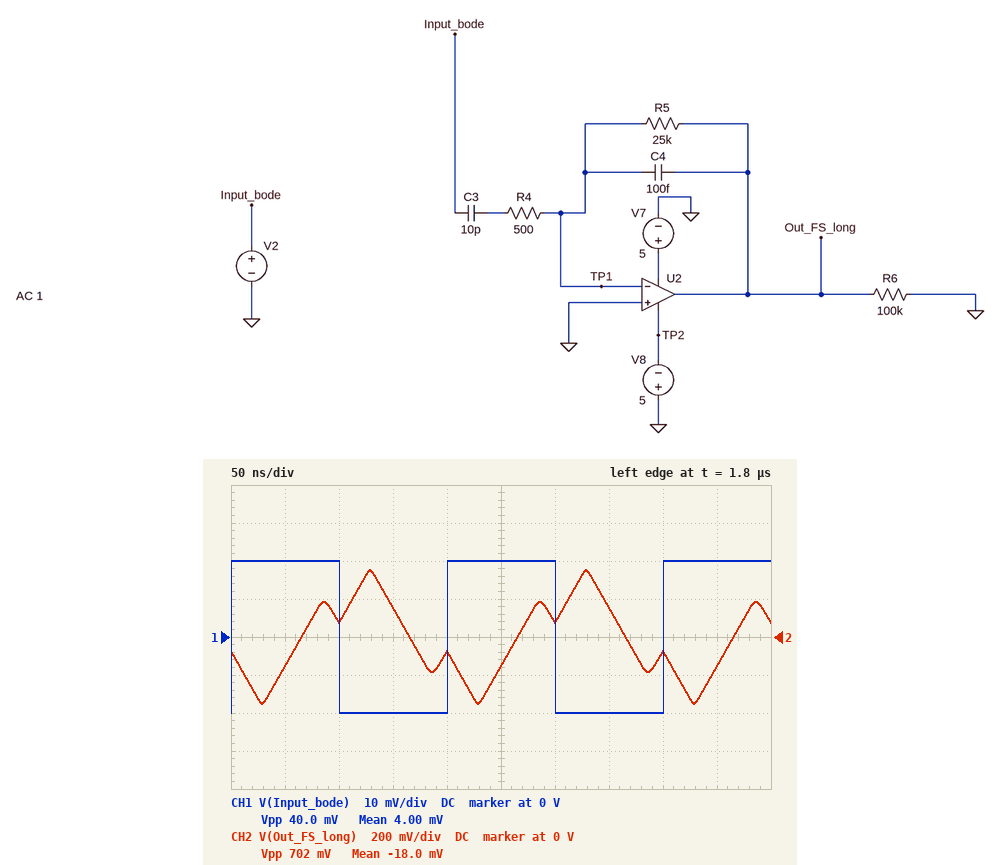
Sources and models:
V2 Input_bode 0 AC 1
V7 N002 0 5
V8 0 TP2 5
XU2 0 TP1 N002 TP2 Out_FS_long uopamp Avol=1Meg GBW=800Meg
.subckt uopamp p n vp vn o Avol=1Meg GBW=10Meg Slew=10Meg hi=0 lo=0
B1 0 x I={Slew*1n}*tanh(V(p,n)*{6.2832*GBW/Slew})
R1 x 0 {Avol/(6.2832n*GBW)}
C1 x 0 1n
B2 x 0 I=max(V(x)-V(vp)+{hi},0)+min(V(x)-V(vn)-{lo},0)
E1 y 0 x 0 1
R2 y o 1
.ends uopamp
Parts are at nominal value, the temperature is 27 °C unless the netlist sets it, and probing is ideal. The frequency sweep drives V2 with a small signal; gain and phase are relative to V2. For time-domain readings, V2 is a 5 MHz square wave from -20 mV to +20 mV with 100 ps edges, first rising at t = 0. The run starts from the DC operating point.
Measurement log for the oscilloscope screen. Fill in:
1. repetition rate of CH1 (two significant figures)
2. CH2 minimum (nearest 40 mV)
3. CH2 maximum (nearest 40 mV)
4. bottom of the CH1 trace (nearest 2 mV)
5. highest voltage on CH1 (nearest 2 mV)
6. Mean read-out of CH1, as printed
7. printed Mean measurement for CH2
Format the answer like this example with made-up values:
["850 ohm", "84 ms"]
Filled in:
["5.0 MHz", "-360 mV", "360 mV", "-20 mV", "20 mV", "4.00 mV", "-18.0 mV"]
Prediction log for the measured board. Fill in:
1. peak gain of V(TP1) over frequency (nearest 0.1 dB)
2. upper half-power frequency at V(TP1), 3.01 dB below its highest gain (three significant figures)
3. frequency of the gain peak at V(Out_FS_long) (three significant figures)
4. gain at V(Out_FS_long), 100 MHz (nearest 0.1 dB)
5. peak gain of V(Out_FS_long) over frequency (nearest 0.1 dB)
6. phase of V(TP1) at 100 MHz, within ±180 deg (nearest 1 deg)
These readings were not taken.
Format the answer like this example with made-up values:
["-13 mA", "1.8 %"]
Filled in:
["-0.6 dB", "2.63 GHz", "20.0 MHz", "16.1 dB", "30.3 dB", "10 deg"]
